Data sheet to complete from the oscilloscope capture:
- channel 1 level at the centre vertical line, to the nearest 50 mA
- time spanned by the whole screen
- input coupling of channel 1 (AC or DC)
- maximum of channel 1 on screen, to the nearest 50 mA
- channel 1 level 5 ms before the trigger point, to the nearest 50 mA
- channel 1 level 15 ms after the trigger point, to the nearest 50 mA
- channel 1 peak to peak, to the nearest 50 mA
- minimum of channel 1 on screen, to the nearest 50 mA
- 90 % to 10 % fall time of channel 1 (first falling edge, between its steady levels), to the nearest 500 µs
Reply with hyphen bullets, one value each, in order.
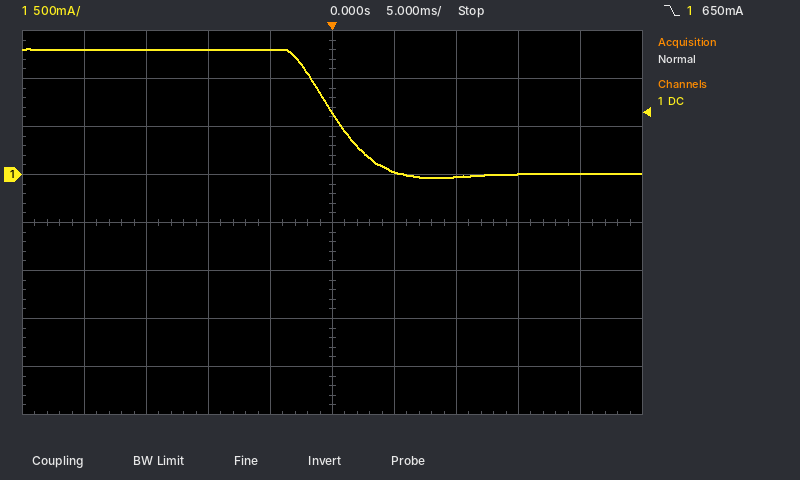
- 650 mA
- 50 ms
- DC
- 1.30 A
- 1.30 A
- 0 mA
- 1.35 A
- -50 mA
- 6.0 ms
